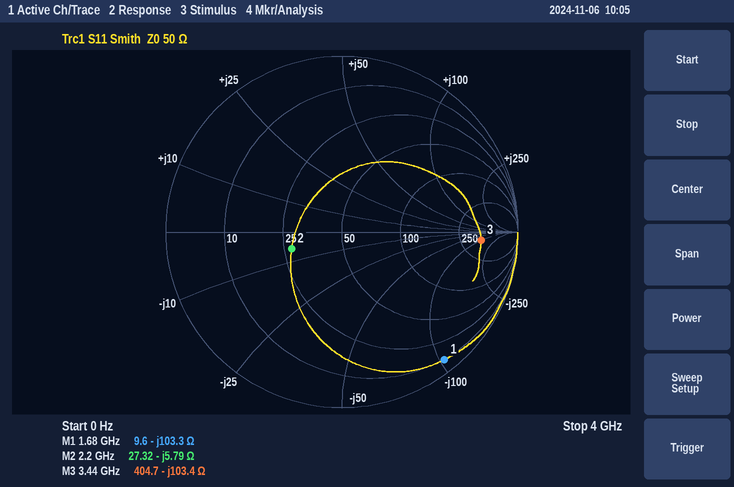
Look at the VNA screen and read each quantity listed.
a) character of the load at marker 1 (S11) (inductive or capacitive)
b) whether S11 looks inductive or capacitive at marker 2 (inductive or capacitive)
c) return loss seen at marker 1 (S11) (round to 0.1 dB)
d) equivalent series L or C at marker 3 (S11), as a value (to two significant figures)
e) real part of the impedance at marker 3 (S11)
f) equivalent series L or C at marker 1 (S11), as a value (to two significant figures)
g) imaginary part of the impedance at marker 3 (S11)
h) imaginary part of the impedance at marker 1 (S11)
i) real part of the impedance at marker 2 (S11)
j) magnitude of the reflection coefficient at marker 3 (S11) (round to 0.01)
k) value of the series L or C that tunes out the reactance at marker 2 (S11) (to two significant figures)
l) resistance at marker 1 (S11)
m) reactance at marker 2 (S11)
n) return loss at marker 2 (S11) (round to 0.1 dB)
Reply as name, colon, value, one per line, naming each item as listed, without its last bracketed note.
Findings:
character of the load at marker 1 (S11): capacitive
whether S11 looks inductive or capacitive at marker 2: capacitive
return loss seen at marker 1 (S11): 0.6 dB
equivalent series L or C at marker 3 (S11), as a value: 450 fF
real part of the impedance at marker 3: 404.7 Ω
equivalent series L or C at marker 1 (S11), as a value: 920 fF
imaginary part of the impedance at marker 3: -103.4 Ω
imaginary part of the impedance at marker 1: -103.3 Ω
real part of the impedance at marker 2: 27.32 Ω
magnitude of the reflection coefficient at marker 3 (S11): 0.79
value of the series L or C that tunes out the reactance at marker 2 (S11): 420 pH
resistance at marker 1: 9.6 Ω
reactance at marker 2: -5.79 Ω
return loss at marker 2 (S11): 10.4 dB
